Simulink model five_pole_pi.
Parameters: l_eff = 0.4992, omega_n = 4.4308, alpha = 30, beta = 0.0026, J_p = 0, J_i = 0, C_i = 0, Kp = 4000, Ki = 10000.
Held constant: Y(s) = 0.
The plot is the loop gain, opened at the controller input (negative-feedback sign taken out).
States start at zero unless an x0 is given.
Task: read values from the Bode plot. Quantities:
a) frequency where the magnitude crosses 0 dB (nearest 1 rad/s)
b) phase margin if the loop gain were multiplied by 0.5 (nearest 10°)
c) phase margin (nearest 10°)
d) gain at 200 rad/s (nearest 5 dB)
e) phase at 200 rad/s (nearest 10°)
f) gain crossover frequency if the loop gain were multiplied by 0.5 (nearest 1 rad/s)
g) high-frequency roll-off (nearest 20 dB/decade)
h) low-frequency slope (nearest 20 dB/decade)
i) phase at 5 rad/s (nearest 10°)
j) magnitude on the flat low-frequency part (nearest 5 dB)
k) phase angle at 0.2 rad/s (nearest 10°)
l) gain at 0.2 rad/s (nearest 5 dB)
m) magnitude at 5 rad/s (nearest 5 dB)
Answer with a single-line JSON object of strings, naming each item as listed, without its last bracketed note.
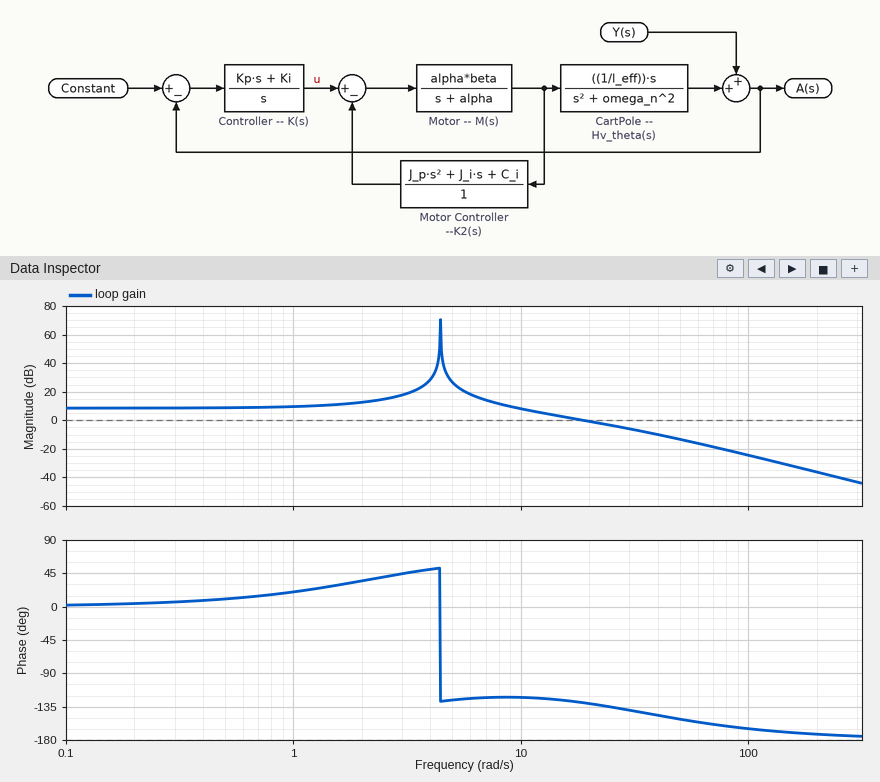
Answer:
{"frequency where the magnitude crosses 0 dB": "19 rad/s", "phase margin if the loop gain were multiplied by 0.5": "60°", "phase margin": "50°", "gain at 200 rad/s": "-35 dB", "phase at 200 rad/s": "-170°", "gain crossover frequency if the loop gain were multiplied by 0.5": "12 rad/s", "high-frequency roll-off": "-40 dB/decade", "low-frequency slope": "0 dB/decade", "phase at 5 rad/s": "-130°", "magnitude on the flat low-frequency part": "10 dB", "phase angle at 0.2 rad/s": "0°", "gain at 0.2 rad/s": "10 dB", "magnitude at 5 rad/s": "25 dB"}
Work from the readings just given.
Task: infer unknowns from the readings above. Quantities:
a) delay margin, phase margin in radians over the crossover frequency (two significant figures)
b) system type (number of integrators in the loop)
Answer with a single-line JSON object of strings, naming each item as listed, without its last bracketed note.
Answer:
{"delay margin, phase margin in radians over the crossover frequency": "0.046 s", "system type": "0"}
